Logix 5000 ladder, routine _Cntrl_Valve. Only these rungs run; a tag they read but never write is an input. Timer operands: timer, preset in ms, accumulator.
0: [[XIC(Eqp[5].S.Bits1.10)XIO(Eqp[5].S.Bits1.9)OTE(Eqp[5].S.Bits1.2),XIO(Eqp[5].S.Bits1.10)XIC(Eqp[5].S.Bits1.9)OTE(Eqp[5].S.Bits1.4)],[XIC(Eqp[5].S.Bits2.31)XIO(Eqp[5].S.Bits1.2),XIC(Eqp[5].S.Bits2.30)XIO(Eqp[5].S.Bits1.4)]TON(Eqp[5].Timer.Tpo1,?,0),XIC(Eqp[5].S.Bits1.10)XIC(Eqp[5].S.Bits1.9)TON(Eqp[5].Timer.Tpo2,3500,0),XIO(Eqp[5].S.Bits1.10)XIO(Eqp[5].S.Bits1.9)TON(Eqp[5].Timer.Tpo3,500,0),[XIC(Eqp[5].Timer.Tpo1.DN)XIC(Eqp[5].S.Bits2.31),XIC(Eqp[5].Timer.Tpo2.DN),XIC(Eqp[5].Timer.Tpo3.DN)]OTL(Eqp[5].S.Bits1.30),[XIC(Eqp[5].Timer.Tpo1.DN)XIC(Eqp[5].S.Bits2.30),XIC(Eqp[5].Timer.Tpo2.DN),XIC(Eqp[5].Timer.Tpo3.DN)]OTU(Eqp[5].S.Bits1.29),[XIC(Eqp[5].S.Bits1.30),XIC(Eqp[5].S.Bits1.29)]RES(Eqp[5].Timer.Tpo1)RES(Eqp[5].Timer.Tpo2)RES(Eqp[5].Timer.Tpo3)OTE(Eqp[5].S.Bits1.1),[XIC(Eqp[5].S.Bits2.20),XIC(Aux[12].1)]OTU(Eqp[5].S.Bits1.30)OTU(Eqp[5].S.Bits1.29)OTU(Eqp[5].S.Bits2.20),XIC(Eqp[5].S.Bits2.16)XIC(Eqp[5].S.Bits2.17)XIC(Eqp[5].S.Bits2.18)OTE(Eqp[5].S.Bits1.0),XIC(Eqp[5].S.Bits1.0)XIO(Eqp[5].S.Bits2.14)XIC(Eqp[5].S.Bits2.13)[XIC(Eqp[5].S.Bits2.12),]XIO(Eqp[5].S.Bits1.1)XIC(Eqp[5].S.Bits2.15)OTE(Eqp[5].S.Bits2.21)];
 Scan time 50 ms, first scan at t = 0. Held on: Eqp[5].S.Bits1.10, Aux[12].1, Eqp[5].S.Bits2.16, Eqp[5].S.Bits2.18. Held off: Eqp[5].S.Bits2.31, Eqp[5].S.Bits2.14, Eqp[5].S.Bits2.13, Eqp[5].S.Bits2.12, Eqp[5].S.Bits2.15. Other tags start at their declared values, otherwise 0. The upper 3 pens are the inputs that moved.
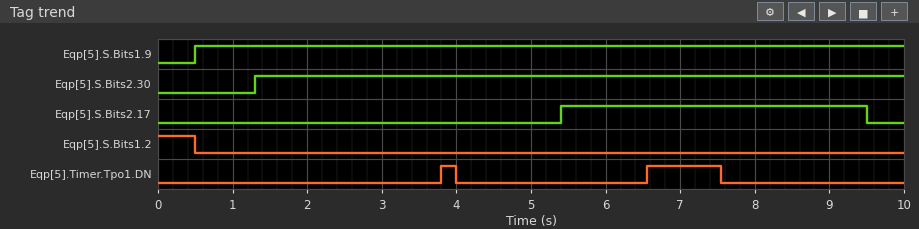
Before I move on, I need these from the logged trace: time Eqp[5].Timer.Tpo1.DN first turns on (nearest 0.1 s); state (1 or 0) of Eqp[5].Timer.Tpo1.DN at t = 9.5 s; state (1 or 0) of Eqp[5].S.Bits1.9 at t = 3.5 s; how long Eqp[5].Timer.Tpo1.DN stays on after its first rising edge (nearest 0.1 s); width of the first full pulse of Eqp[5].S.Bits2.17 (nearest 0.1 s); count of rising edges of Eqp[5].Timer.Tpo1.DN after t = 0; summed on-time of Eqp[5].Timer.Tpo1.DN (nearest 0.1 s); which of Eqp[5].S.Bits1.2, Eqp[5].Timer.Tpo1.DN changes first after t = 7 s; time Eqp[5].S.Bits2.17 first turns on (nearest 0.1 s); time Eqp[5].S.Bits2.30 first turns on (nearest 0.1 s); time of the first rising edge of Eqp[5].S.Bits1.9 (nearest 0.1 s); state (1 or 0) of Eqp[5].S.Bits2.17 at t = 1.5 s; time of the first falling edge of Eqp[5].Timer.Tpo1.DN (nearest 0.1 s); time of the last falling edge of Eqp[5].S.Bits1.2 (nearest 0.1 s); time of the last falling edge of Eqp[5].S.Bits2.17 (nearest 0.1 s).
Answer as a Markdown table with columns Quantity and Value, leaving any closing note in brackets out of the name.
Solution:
| Quantity | Value |
|---|---|
| time Eqp[5].Timer.Tpo1.DN first turns on | 3.8 s |
| state (1 or 0) of Eqp[5].Timer.Tpo1.DN at t = 9.5 s | 0 |
| state (1 or 0) of Eqp[5].S.Bits1.9 at t = 3.5 s | 1 |
| how long Eqp[5].Timer.Tpo1.DN stays on after its first rising edge | 0.2 s |
| width of the first full pulse of Eqp[5].S.Bits2.17 | 4.1 s |
| count of rising edges of Eqp[5].Timer.Tpo1.DN after t = 0 | 2 |
| summed on-time of Eqp[5].Timer.Tpo1.DN | 1.2 s |
| which of Eqp[5].S.Bits1.2, Eqp[5].Timer.Tpo1.DN changes first after t = 7 s | Eqp[5].Timer.Tpo1.DN |
| time Eqp[5].S.Bits2.17 first turns on | 5.4 s |
| time Eqp[5].S.Bits2.30 first turns on | 1.3 s |
| time of the first rising edge of Eqp[5].S.Bits1.9 | 0.5 s |
| state (1 or 0) of Eqp[5].S.Bits2.17 at t = 1.5 s | 0 |
| time of the first falling edge of Eqp[5].Timer.Tpo1.DN | 4.0 s |
| time of the last falling edge of Eqp[5].S.Bits1.2 | 0.5 s |
| time of the last falling edge of Eqp[5].S.Bits2.17 | 9.5 s |
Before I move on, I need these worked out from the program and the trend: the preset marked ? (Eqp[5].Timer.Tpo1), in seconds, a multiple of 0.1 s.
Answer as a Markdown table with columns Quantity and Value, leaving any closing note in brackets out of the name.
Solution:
| Quantity | Value |
|---|---|
| the preset marked ? (Eqp[5].Timer.Tpo1), in seconds, a multiple of 0.1 s | 2.5 s |
